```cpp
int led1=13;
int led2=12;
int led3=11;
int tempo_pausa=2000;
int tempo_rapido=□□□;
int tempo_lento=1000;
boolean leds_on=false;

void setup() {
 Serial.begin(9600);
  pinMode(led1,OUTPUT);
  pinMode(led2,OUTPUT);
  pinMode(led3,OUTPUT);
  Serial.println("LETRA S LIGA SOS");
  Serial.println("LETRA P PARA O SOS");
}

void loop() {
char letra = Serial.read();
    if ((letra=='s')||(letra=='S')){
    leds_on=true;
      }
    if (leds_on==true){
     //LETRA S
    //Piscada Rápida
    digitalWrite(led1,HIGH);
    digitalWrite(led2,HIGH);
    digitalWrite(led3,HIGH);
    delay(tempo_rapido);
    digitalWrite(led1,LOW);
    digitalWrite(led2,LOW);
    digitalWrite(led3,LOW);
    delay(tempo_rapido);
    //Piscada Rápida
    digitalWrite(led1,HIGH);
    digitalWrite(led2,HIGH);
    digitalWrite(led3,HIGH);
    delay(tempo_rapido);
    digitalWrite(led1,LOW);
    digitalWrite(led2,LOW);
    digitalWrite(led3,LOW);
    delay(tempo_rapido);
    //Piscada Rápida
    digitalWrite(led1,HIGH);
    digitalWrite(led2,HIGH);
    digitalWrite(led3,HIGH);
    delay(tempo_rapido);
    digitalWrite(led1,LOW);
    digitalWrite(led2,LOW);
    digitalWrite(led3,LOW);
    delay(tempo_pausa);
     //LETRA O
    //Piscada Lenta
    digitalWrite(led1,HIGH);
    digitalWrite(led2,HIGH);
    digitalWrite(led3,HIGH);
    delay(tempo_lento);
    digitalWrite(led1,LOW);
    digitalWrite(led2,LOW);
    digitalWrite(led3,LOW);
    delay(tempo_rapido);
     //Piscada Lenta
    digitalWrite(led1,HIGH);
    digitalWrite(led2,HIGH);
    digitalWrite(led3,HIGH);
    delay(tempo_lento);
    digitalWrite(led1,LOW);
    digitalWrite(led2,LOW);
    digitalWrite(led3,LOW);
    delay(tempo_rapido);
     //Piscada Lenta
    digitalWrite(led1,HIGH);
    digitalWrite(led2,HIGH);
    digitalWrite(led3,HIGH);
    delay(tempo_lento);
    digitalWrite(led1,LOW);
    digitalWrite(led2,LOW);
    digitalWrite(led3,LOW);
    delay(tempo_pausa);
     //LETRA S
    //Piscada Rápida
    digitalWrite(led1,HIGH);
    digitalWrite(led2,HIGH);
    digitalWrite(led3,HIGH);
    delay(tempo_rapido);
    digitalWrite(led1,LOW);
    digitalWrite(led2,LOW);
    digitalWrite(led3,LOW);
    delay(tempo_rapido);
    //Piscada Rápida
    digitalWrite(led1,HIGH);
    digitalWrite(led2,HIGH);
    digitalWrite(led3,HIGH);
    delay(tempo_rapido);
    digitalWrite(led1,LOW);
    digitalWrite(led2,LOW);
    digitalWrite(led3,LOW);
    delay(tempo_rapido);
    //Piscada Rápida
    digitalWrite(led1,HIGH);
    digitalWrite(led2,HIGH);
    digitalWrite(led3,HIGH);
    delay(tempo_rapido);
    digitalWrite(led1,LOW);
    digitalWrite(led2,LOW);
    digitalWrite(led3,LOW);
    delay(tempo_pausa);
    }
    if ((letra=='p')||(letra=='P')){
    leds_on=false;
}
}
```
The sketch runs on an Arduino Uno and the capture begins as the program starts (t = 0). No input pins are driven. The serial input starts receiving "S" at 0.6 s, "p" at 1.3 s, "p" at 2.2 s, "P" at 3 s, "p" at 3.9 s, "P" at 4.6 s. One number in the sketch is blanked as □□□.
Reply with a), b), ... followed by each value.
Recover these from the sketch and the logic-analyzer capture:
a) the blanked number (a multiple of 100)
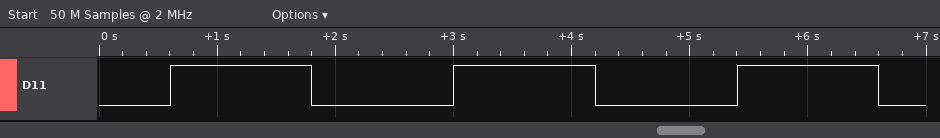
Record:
a) 1200
